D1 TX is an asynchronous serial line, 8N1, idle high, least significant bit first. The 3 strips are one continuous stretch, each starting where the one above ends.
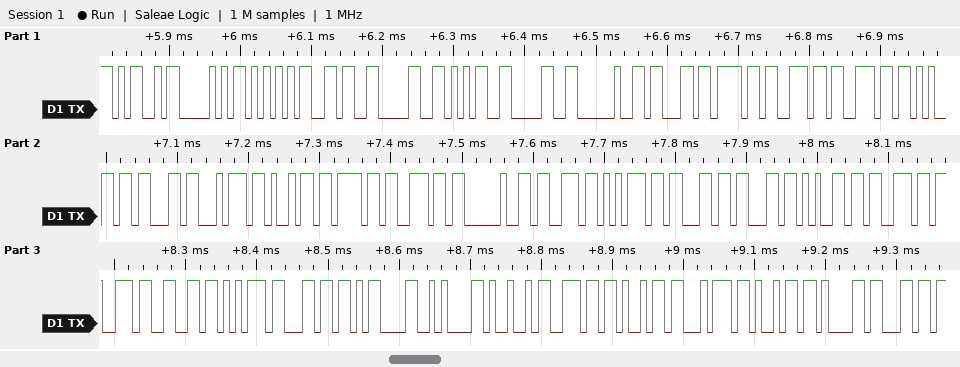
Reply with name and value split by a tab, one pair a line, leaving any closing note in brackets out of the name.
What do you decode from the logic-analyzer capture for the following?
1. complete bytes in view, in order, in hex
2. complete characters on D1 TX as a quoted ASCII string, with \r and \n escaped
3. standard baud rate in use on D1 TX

complete bytes in view, in order, in hex	4D 50 55 36 30 35 30 20 63 6F 6E 6E 65 63 74 69 6F 6E 20 73 75 63 63 65 73 73 66 75 6C 0D 0A 49 6E 69 74 69 61 6C
complete characters on D1 TX as a quoted ASCII string, with \r and \n escaped	"MPU6050 connection successful\r\nInitial"
standard baud rate in use on D1 TX	115200 baud
